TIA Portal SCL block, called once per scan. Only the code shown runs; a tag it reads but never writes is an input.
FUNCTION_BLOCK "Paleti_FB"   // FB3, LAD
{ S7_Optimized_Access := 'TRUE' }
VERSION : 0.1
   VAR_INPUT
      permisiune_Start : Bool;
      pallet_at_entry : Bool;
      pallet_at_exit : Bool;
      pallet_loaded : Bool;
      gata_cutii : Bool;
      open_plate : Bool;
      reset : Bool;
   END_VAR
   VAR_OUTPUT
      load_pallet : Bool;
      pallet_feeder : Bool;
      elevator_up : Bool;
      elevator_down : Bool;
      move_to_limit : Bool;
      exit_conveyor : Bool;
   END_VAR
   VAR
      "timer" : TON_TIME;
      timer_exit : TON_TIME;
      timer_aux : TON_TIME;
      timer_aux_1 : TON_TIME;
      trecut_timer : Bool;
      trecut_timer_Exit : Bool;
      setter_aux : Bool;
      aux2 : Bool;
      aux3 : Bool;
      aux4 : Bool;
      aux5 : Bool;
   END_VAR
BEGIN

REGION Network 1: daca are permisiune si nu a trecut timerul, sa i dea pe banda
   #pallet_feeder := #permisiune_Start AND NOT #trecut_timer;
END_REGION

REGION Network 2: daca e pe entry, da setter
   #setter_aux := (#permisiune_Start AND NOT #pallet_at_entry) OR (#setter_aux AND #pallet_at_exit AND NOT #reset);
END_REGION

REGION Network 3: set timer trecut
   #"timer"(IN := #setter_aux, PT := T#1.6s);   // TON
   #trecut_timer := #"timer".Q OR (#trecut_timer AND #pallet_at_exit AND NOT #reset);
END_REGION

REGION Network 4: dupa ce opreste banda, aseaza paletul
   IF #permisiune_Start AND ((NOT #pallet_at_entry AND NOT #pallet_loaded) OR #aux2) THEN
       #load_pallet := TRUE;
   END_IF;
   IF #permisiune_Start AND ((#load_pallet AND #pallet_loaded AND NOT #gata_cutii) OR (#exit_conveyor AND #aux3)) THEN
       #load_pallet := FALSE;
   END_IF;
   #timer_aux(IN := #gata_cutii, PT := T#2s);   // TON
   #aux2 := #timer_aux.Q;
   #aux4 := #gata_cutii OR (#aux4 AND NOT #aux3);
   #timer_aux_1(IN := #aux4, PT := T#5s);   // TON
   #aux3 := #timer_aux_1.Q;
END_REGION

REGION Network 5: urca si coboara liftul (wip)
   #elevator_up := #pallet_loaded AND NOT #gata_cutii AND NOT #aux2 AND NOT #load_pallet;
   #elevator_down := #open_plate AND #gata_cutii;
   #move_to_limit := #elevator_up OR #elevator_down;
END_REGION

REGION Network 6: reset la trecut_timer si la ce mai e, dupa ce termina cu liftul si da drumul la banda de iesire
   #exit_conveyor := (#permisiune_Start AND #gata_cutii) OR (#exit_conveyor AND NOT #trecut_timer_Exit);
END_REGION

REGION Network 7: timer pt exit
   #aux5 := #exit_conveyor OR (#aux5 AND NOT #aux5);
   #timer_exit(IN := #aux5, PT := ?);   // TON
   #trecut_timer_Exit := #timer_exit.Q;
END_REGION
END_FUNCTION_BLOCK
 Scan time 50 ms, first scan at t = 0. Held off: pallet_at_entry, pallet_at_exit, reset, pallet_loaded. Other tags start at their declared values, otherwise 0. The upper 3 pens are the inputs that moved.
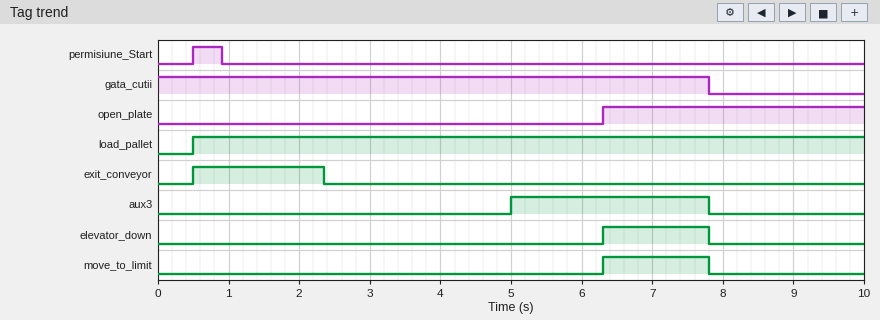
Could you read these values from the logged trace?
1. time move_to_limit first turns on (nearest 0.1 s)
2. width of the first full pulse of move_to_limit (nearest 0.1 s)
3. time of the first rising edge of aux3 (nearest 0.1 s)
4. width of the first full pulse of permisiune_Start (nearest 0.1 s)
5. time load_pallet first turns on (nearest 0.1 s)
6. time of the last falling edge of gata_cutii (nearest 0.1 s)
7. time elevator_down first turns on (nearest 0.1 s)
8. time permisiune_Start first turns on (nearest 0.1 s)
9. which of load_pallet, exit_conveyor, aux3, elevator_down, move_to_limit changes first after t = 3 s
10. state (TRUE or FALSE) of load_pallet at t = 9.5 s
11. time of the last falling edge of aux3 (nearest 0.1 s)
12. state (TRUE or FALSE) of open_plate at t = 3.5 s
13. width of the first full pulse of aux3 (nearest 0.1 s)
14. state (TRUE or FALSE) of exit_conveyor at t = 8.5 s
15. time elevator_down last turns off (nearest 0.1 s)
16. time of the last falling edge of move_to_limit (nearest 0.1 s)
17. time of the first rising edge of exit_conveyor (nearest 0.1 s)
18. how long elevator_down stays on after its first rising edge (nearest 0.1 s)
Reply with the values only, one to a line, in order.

6.3 s
1.5 s
5.0 s
0.4 s
0.5 s
7.8 s
6.3 s
0.5 s
aux3
TRUE
7.8 s
FALSE
2.8 s
FALSE
7.8 s
7.8 s
0.5 s
1.5 s
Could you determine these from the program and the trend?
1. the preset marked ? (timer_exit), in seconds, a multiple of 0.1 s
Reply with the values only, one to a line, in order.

1.8 s
